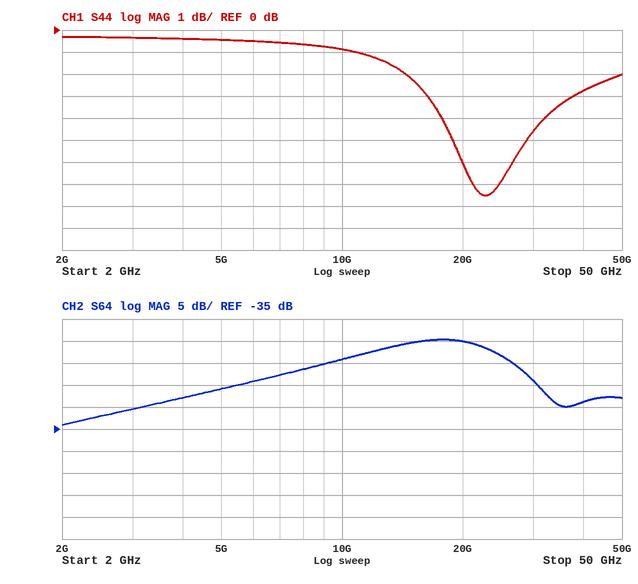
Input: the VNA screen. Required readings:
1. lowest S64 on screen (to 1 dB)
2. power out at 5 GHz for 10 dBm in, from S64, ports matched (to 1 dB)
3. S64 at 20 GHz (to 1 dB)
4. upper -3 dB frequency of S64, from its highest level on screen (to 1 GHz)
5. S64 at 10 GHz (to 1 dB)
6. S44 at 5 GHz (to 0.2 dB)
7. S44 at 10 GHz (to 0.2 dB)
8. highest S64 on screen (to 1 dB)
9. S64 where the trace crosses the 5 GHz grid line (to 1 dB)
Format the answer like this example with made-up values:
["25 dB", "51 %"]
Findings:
["-34 dB", "-16 dBm", "-15 dB", "24 GHz", "-19 dB", "-0.4 dB", "-0.8 dB", "-15 dB", "-26 dB"]
